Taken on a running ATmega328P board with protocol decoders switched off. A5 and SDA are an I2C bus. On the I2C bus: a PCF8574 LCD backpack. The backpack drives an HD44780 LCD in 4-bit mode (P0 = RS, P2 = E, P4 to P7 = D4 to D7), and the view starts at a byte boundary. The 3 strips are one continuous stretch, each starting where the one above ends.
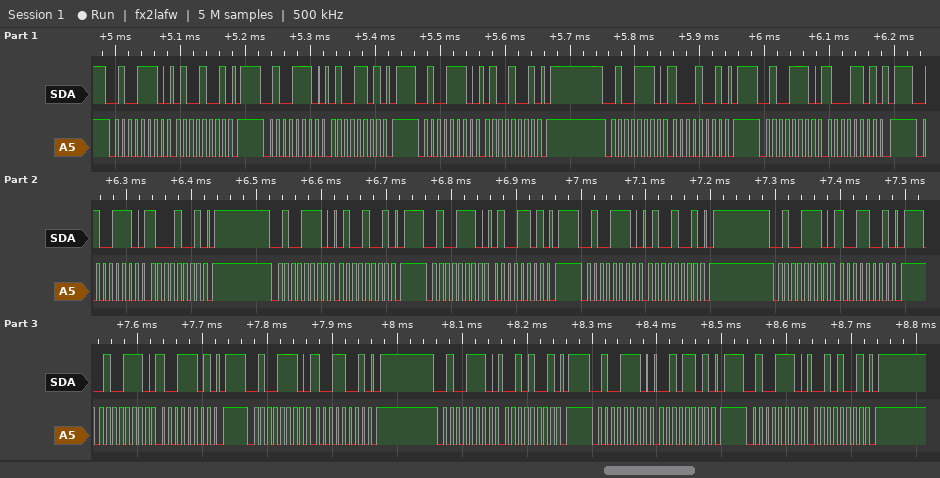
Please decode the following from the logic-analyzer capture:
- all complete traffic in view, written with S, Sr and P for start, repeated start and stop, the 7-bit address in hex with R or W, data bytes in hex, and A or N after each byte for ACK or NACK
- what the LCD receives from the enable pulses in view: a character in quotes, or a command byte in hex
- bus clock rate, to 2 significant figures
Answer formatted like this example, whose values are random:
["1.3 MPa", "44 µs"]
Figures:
["S 27W A 49 A P S 27W A 4D A P S 27W A 49 A P S 27W A 89 A P S 27W A 8D A P S 27W A 89 A P S 27W A 49 A P S 27W A 4D A P S 27W A 49 A P S 27W A 99 A P S 27W A 9D A P S 27W A 99 A P S 27W A 29 A P S 27W A 2D A P S 27W A 29 A P", "'H' 'I'", "100 kHz"]
